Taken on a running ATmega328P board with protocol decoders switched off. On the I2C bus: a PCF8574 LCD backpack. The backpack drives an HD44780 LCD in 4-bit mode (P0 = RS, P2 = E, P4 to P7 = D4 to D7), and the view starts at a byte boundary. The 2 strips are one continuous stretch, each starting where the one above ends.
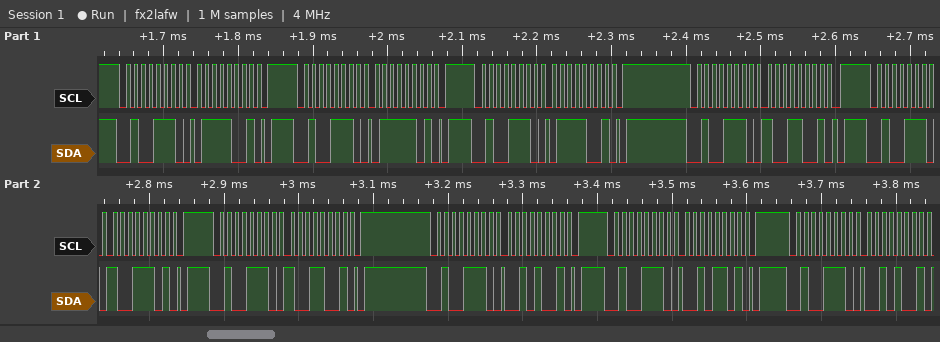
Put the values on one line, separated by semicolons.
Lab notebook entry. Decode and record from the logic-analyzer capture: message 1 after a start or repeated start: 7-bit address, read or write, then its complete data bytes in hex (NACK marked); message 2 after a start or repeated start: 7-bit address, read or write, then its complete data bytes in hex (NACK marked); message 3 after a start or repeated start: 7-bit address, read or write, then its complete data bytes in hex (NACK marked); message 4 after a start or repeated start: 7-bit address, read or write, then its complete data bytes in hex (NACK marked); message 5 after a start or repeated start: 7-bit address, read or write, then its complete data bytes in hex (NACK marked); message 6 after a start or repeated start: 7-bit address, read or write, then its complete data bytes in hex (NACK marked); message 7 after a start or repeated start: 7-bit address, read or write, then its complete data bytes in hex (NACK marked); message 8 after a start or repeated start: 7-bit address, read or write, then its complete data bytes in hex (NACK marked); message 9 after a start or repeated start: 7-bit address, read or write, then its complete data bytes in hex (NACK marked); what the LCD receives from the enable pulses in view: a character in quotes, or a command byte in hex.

0x27 write: 79; 0x27 write: 7D; 0x27 write: 79; 0x27 write: 99; 0x27 write: 9D; 0x27 write: 99; 0x27 write: 29; 0x27 write: 2D; 0x27 write: 29; 'y'
